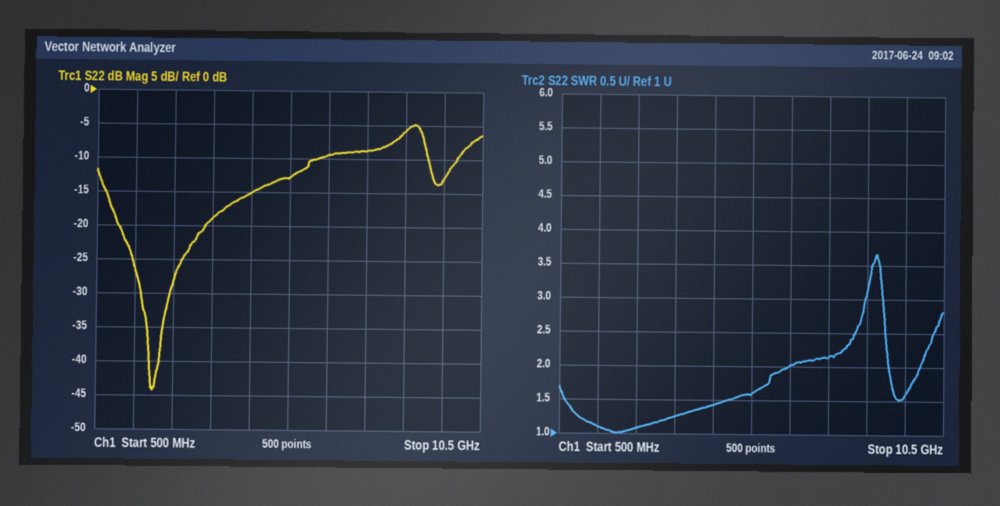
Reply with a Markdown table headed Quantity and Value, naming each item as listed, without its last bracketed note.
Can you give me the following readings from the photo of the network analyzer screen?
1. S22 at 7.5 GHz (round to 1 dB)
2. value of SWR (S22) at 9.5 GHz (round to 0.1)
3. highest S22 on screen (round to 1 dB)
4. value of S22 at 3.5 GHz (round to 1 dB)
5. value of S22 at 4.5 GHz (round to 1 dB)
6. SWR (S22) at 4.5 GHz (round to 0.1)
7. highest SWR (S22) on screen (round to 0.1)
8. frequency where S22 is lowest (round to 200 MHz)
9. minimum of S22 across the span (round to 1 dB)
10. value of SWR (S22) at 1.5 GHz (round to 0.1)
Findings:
| Quantity | Value |
|---|---|
| S22 at 7.5 GHz | -9 dB |
| value of SWR (S22) at 9.5 GHz | 1.6 |
| highest S22 on screen | -5 dB |
| value of S22 at 3.5 GHz | -19 dB |
| value of S22 at 4.5 GHz | -15 dB |
| SWR (S22) at 4.5 GHz | 1.4 |
| highest SWR (S22) on screen | 3.7 |
| frequency where S22 is lowest | 2.0 GHz |
| minimum of S22 across the span | -44 dB |
| value of SWR (S22) at 1.5 GHz | 1.1 |
